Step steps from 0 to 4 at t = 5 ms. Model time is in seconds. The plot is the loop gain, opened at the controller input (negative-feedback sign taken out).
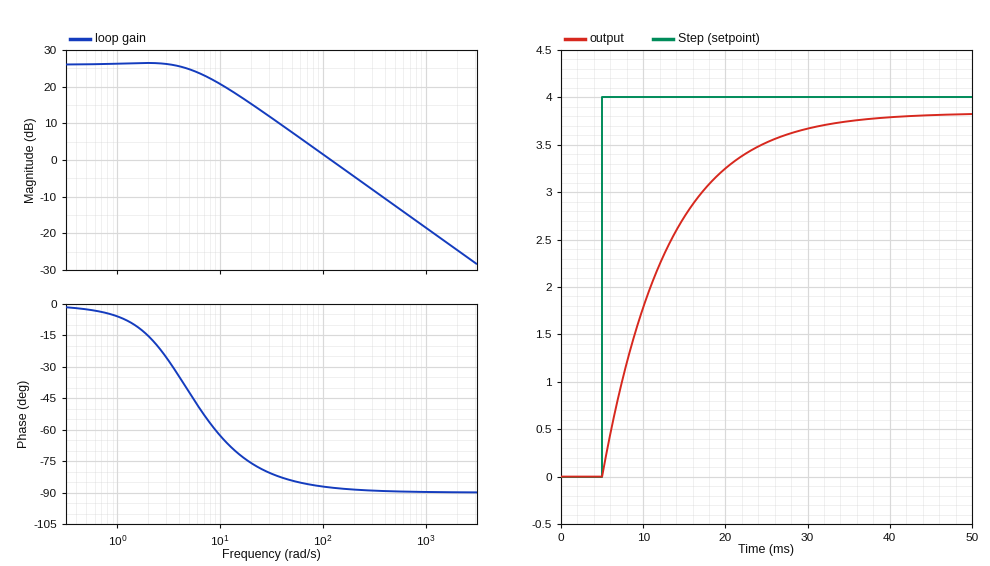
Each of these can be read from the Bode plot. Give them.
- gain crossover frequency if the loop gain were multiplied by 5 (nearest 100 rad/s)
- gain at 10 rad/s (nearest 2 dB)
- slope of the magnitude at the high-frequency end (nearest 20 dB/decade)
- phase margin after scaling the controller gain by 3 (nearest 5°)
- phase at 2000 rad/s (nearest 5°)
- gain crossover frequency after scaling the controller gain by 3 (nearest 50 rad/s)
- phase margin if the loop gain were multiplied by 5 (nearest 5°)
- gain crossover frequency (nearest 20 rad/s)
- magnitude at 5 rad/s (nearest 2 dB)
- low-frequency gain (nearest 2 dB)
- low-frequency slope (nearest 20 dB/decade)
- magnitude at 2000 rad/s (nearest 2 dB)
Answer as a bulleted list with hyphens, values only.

- 600 rad/s
- 20 dB
- -20 dB/decade
- 90°
- -90°
- 350 rad/s
- 90°
- 120 rad/s
- 24 dB
- 26 dB
- 0 dB/decade
- -24 dB
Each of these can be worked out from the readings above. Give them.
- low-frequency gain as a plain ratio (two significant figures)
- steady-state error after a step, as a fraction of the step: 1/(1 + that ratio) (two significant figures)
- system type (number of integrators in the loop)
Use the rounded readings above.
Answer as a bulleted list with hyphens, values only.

- 20
- 0.048
- 0
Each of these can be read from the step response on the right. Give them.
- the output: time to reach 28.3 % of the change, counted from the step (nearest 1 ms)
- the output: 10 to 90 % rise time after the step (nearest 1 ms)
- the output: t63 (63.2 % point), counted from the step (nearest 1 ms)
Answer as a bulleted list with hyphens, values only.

- 3 ms
- 17 ms
- 8 ms
